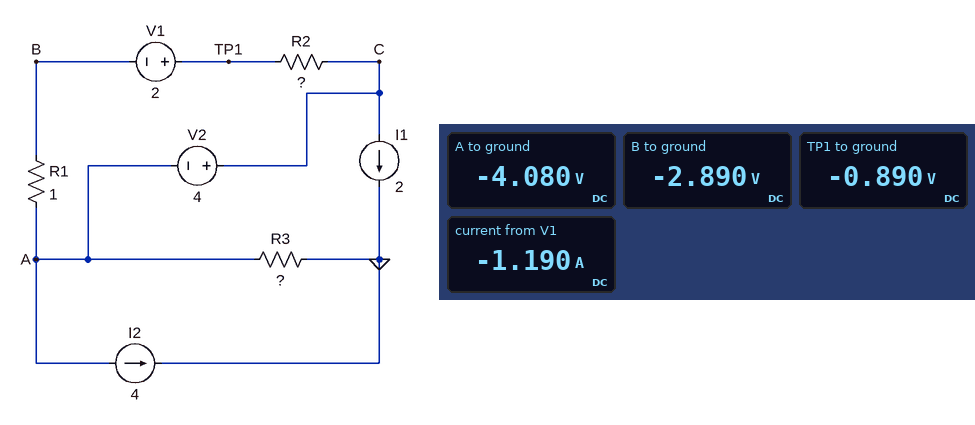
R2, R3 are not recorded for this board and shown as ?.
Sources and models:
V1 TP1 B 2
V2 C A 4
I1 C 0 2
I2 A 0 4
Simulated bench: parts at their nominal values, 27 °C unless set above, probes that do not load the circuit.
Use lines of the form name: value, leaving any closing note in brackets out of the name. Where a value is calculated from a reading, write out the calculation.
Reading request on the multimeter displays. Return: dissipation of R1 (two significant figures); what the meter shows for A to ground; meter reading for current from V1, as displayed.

dissipation of R1: (-2.89 V - (-4.08 V))^2 / 1 Ω = 1.4 W
what the meter shows for A to ground: -4.080 V
meter reading for current from V1, as displayed: -1.190 A
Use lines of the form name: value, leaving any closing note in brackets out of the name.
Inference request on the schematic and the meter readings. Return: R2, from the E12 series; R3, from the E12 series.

R2, from the E12 series: 0.68 Ω
R3, from the E12 series: 0.68 Ω
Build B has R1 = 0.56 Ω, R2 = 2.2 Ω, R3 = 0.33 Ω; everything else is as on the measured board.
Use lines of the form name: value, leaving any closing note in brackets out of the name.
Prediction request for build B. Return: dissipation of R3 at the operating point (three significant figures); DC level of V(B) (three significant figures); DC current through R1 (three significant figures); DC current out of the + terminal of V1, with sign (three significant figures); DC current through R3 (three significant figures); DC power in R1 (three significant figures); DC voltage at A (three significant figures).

dissipation of R3 at the operating point: 11.9 W
DC level of V(B): -1.57 V
DC current through R1: 725 mA
DC current out of the + terminal of V1, with sign: -725 mA
DC current through R3: 6.00 A
DC power in R1: 294 mW
DC voltage at A: -1.98 V
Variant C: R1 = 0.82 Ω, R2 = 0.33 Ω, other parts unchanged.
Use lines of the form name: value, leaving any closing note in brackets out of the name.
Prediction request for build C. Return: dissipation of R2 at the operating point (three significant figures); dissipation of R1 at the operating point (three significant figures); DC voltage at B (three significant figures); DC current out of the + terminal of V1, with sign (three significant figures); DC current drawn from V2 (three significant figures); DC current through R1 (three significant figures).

dissipation of R2 at the operating point: 998 mW
dissipation of R1 at the operating point: 2.48 W
DC voltage at B: -2.65 V
DC current out of the + terminal of V1, with sign: -1.74 A
DC current drawn from V2: 3.74 A
DC current through R1: 1.74 A
